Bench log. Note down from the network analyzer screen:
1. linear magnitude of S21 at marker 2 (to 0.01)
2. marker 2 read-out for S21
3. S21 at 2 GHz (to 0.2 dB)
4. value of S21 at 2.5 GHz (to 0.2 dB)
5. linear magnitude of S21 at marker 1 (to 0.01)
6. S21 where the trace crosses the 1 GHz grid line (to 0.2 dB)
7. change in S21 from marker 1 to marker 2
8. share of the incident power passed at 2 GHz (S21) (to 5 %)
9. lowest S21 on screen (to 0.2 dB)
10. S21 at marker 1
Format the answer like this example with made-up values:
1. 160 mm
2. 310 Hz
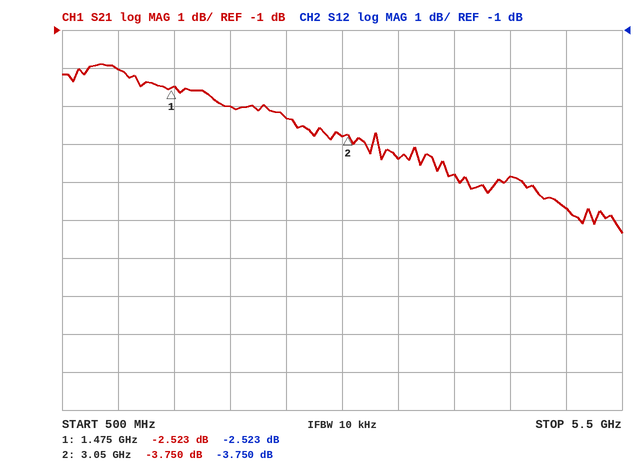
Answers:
1. 0.65
2. -3.750 dB
3. -3.0 dB
4. -3.4 dB
5. 0.75
6. -2.0 dB
7. -1.227 dB
8. 50 %
9. -6.4 dB
10. -2.523 dB
